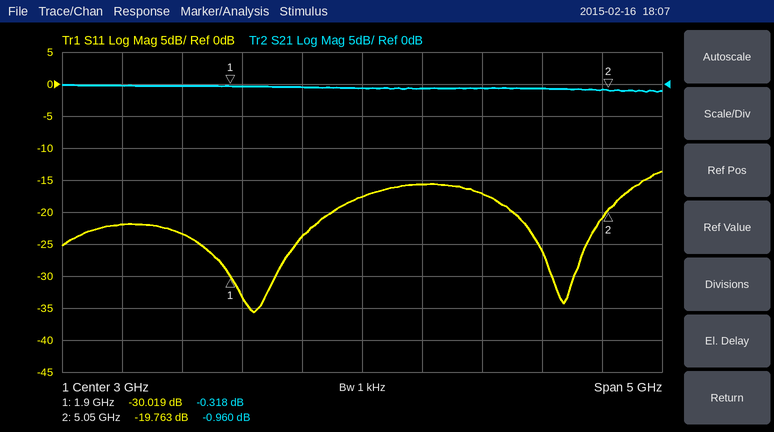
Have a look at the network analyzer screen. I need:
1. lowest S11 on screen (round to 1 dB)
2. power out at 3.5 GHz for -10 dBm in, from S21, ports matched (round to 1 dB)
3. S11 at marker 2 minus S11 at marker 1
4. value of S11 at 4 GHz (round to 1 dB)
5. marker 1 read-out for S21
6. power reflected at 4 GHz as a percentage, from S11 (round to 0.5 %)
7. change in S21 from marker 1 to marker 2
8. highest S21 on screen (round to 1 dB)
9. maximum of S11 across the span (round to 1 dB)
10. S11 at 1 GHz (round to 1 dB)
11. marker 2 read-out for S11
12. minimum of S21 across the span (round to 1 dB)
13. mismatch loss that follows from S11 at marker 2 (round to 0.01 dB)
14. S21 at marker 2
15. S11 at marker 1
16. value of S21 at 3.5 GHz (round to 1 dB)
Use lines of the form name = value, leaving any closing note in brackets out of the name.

lowest S11 on screen = -36 dB
power out at 3.5 GHz for -10 dBm in, from S21, ports matched = -11 dBm
S11 at marker 2 minus S11 at marker 1 = 10.256 dB
value of S11 at 4 GHz = -17 dB
marker 1 read-out for S21 = -0.318 dB
power reflected at 4 GHz as a percentage, from S11 = 2.0 %
change in S21 from marker 1 to marker 2 = -0.642 dB
highest S21 on screen = 0 dB
maximum of S11 across the span = -14 dB
S11 at 1 GHz = -22 dB
marker 2 read-out for S11 = -19.763 dB
minimum of S21 across the span = -1 dB
mismatch loss that follows from S11 at marker 2 = 0.05 dB
S21 at marker 2 = -0.960 dB
S11 at marker 1 = -30.019 dB
value of S21 at 3.5 GHz = -1 dB
